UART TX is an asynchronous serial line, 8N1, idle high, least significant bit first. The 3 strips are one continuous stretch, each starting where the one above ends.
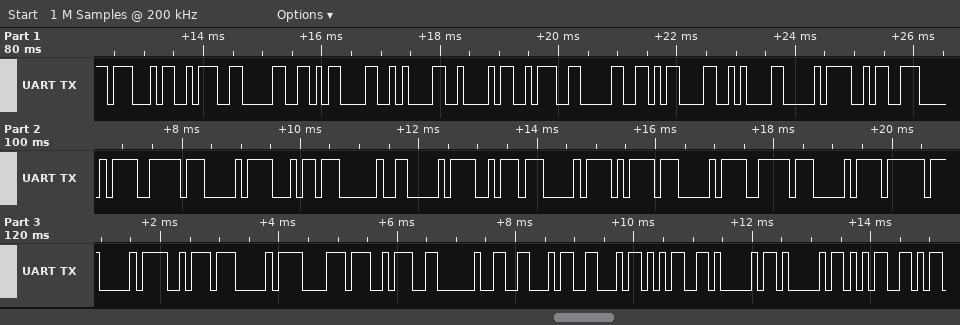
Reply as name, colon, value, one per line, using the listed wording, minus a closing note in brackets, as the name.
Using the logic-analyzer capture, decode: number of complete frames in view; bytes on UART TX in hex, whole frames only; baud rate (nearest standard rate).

number of complete frames in view: 37
bytes on UART TX in hex, whole frames only: 0x47 0x3A 0x30 0x0D 0x0A 0x42 0x3A 0x30 0x0D 0x0A 0xD0 0x9A 0xD0 0xBE 0xD0 0xB4 0x20 0xD0 0xBA 0xD0 0xBD 0xD0 0xBE 0xD0 0xBF 0xD0 0xBA 0xD0 0xB8 0x3A 0x20 0x46 0x46 0x35 0x41 0x41 0x35
baud rate: 9600 baud
